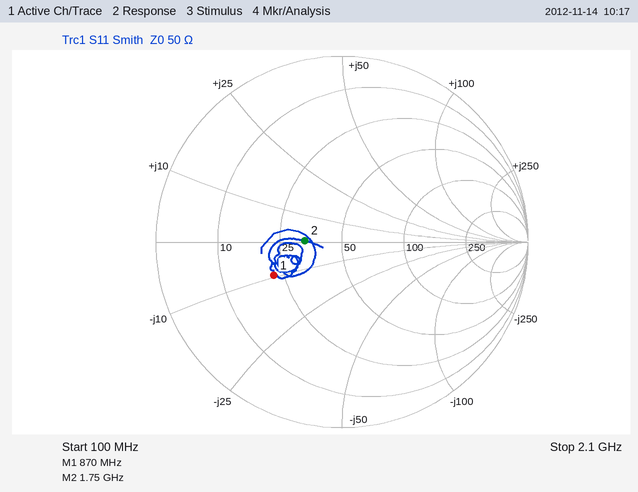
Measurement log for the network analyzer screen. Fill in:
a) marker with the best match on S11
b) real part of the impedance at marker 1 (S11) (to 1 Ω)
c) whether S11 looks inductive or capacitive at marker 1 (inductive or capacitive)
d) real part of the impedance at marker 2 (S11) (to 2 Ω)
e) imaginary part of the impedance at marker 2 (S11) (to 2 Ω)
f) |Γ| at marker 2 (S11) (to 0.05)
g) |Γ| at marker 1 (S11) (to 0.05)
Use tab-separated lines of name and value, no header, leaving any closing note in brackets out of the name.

marker with the best match on S11	marker 2
real part of the impedance at marker 1 (S11)	22 Ω
whether S11 looks inductive or capacitive at marker 1	capacitive
real part of the impedance at marker 2 (S11)	34 Ω
imaginary part of the impedance at marker 2 (S11)	0 Ω
|Γ| at marker 2 (S11)	0.20
|Γ| at marker 1 (S11)	0.40
